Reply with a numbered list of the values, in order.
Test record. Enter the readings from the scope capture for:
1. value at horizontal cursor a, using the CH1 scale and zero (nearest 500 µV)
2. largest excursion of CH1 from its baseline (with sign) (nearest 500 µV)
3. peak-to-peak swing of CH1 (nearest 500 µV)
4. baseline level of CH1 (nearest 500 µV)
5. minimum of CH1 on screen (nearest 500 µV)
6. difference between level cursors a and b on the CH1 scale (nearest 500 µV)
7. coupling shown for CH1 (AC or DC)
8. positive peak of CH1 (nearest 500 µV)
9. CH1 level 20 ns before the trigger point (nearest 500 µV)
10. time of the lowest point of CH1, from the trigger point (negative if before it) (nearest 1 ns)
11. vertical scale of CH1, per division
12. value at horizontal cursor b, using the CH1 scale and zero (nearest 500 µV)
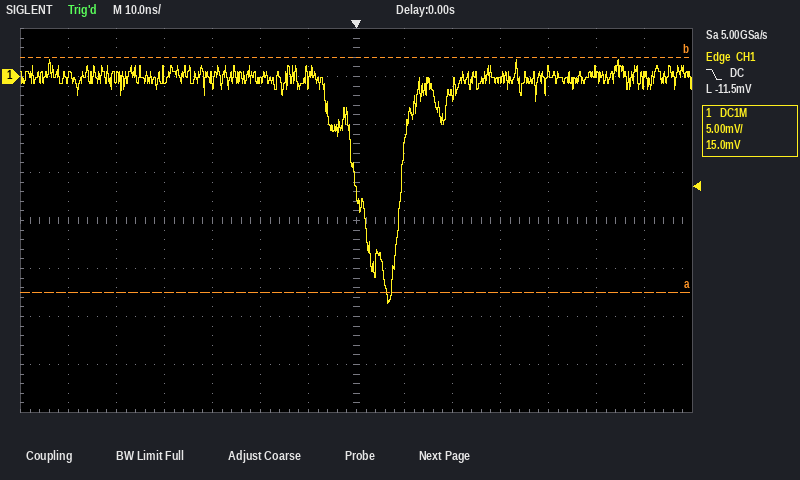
1. -22.5 mV
2. -23.5 mV
3. 25.5 mV
4. 0.0 mV
5. -23.5 mV
6. 24.5 mV
7. DC
8. 2.0 mV
9. -500 µV
10. +7 ns
11. 5 mV
12. 2.0 mV
